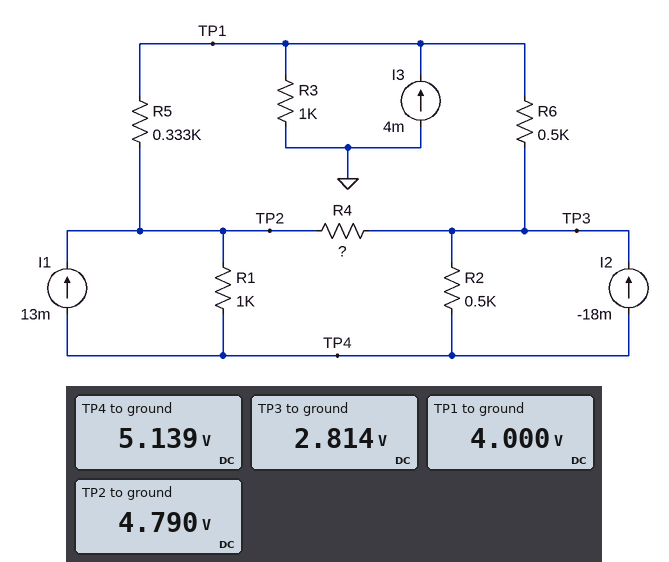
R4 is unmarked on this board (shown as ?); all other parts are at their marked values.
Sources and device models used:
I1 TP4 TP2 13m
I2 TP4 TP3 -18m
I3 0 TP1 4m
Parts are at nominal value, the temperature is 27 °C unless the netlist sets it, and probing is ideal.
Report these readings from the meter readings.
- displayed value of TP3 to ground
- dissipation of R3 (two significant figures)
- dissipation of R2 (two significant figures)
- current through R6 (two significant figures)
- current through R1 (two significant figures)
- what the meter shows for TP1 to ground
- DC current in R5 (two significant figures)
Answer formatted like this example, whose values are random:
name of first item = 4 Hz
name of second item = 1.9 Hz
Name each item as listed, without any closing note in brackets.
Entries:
displayed value of TP3 to ground = 2.814 V
dissipation of R3 = 16 mW
dissipation of R2 = 11 mW
current through R6 = 2.4 mA
current through R1 = 350 µA
what the meter shows for TP1 to ground = 4.000 V
DC current in R5 = 2.4 mA
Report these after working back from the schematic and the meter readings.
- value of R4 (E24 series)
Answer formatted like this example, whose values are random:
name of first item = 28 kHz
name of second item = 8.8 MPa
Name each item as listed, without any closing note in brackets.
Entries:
value of R4 = 180 Ω
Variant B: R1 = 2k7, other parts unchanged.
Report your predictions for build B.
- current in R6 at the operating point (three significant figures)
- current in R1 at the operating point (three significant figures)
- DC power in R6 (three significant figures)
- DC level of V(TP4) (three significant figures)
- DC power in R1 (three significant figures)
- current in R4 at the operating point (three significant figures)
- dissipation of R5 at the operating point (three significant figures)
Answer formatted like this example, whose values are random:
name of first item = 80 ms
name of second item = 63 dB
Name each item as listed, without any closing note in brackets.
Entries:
current in R6 at the operating point = 2.34 mA
current in R1 at the operating point = 172 µA
DC power in R6 = 2.74 mW
DC level of V(TP4) = 5.24 V
DC power in R1 = 79.9 µW
current in R4 at the operating point = 10.8 mA
dissipation of R5 at the operating point = 1.82 mW
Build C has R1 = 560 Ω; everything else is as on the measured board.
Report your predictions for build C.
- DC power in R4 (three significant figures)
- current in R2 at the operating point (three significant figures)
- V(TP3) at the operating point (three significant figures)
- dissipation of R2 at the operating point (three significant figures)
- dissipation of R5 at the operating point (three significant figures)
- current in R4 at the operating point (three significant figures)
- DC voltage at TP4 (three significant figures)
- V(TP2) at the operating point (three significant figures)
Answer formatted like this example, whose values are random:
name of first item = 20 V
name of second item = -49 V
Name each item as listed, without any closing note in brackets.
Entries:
DC power in R4 = 22.1 mW
current in R2 at the operating point = 4.52 mA
V(TP3) at the operating point = 2.80 V
dissipation of R2 at the operating point = 10.2 mW
dissipation of R5 at the operating point = 1.91 mW
current in R4 at the operating point = 11.1 mA
DC voltage at TP4 = 5.06 V
V(TP2) at the operating point = 4.80 V
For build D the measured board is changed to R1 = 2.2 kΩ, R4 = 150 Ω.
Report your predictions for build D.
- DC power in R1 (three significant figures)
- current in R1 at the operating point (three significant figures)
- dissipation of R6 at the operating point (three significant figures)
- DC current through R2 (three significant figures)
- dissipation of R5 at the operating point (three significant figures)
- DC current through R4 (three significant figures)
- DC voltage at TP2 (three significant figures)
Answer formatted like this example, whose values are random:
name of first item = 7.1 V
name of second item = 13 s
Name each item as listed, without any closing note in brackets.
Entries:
DC power in R1 = 198 µW
current in R1 at the operating point = 300 µA
dissipation of R6 at the operating point = 2.06 mW
DC current through R2 = 4.70 mA
dissipation of R5 at the operating point = 1.37 mW
DC current through R4 = 11.3 mA
DC voltage at TP2 = 4.68 V
